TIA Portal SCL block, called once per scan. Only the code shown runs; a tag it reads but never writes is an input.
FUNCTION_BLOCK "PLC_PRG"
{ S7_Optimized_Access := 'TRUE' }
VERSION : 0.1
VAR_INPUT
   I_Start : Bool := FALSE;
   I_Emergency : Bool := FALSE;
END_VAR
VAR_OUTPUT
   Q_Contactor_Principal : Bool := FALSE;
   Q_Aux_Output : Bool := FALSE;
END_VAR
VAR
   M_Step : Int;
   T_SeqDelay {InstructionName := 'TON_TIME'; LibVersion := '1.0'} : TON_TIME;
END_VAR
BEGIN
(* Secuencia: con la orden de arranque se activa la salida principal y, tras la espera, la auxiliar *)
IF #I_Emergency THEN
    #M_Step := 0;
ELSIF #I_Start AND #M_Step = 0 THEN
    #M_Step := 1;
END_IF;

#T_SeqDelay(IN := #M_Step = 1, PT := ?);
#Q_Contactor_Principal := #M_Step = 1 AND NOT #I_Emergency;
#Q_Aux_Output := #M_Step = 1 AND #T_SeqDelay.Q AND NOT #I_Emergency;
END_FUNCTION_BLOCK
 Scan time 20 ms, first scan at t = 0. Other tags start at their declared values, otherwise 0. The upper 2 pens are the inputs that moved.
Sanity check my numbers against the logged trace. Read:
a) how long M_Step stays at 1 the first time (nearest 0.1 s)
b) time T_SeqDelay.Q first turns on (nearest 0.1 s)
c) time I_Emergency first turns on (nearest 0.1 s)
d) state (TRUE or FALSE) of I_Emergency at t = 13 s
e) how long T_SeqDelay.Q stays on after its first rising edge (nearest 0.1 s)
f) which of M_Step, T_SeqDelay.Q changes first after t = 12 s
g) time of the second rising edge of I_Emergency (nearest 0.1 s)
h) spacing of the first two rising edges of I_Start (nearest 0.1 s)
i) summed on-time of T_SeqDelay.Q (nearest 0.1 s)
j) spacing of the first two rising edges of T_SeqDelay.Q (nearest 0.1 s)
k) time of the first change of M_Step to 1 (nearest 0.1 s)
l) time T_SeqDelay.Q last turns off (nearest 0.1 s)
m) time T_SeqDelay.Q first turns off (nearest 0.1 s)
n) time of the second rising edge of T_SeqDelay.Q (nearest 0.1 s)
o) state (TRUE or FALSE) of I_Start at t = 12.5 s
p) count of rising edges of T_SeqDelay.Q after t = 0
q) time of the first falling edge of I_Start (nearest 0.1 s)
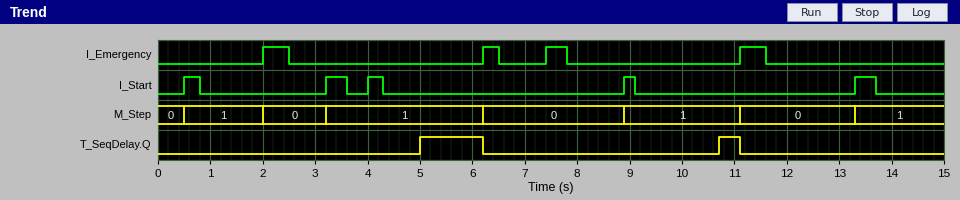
1.5 s
5.0 s
2.0 s
FALSE
1.2 s
M_Step
6.2 s
2.7 s
1.6 s
5.7 s
0.5 s
11.1 s
6.2 s
10.7 s
FALSE
2
0.8 s
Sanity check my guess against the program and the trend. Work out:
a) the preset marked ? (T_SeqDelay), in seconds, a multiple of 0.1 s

1.8 s
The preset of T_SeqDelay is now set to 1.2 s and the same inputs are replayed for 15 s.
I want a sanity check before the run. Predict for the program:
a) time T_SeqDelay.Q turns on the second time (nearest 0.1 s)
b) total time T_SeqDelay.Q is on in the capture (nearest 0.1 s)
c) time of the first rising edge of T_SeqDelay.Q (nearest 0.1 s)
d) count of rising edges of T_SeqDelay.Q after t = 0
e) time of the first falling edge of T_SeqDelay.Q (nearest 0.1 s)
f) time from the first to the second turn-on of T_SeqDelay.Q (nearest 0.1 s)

4.4 s
3.6 s
1.7 s
4
2.0 s
2.7 s
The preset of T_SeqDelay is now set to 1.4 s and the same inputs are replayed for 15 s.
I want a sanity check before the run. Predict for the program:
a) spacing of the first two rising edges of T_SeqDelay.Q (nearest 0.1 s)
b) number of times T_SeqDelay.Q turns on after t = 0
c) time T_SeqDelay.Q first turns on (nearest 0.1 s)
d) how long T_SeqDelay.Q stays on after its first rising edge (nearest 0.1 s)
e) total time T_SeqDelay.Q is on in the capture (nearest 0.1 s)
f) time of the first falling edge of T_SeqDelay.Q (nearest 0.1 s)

2.7 s
4
1.9 s
0.1 s
2.8 s
2.0 s
